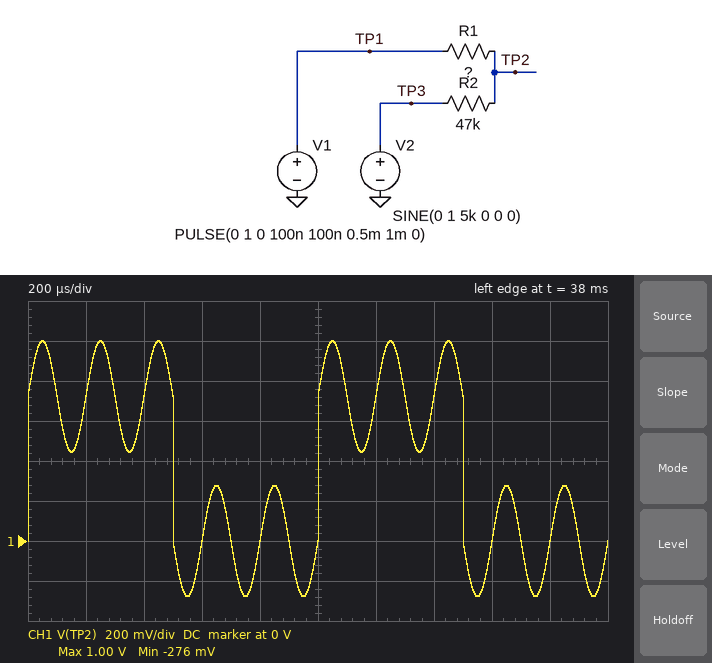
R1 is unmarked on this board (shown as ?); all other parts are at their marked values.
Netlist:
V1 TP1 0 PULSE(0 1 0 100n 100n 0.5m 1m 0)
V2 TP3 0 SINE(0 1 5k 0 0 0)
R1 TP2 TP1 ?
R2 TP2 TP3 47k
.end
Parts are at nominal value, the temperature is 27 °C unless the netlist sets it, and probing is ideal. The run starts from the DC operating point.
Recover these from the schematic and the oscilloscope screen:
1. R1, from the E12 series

18 kΩ
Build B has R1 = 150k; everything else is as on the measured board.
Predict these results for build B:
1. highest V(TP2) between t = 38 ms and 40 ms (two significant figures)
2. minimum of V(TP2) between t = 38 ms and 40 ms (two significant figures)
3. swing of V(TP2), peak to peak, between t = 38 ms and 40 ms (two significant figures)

1.0 V
-760 mV
1.8 V
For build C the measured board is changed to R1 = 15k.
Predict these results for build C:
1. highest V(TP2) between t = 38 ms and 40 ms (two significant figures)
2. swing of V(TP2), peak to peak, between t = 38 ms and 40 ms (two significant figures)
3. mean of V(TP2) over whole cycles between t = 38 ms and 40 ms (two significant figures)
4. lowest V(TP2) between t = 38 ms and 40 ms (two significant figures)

1.0 V
1.2 V
380 mV
-240 mV
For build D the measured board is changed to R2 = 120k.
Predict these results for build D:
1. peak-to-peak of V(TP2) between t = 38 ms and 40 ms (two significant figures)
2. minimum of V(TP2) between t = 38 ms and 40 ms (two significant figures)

1.1 V
-130 mV
